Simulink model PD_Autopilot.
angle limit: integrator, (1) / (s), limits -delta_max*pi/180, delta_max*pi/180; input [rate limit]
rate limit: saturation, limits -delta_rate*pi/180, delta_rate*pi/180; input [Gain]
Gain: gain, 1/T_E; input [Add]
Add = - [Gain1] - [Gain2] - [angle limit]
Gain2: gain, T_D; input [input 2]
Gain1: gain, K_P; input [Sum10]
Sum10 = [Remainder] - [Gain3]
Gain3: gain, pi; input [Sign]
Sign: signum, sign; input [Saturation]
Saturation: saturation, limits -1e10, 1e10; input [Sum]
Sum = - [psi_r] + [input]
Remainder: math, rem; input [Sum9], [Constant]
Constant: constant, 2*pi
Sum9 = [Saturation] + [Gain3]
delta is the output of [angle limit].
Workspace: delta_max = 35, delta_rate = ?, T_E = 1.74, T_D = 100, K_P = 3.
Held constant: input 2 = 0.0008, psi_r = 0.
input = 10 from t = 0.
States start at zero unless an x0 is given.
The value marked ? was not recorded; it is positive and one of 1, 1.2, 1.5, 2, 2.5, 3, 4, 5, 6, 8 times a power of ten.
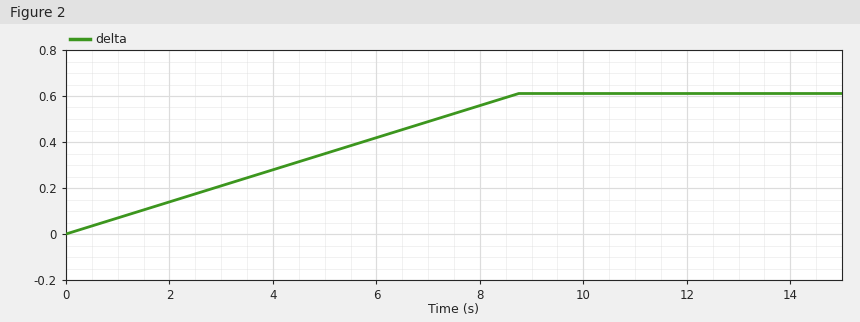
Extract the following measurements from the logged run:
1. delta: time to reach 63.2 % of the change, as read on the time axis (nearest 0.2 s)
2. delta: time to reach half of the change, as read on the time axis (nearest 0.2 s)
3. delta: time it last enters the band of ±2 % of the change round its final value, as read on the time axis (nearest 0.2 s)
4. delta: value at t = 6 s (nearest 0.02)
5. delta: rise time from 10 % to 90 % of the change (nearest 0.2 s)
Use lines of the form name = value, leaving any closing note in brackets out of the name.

delta: time to reach 63.2 % of the change, as read on the time axis = 5.6 s
delta: time to reach half of the change, as read on the time axis = 4.4 s
delta: time it last enters the band of ±2 % of the change round its final value, as read on the time axis = 8.6 s
delta: value at t = 6 s = 0.42
delta: rise time from 10 % to 90 % of the change = 7.0 s
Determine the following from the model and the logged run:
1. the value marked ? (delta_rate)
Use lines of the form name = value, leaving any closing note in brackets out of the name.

the value marked ? = 4
